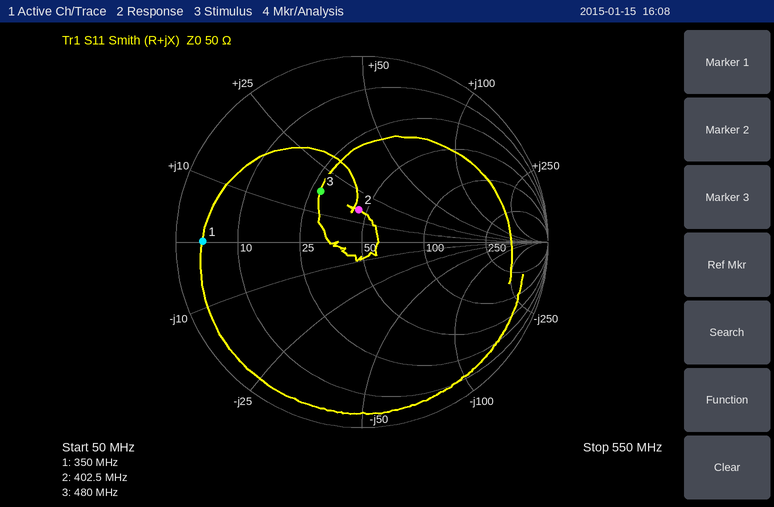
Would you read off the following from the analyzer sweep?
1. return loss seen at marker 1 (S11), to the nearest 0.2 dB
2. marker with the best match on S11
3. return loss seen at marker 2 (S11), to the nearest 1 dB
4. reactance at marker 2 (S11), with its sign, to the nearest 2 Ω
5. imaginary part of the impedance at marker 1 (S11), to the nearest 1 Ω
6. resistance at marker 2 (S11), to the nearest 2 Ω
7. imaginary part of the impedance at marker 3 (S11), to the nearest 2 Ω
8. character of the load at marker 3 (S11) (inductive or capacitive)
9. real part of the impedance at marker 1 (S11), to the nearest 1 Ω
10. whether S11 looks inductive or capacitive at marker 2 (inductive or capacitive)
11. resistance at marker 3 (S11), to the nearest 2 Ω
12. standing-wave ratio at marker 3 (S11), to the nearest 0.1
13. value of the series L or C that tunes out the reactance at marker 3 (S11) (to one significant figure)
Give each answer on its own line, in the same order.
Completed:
1.4 dB
marker 2
15 dB
+16 Ω
0 Ω
46 Ω
+18 Ω
inductive
4 Ω
inductive
28 Ω
2.1
20 pF
